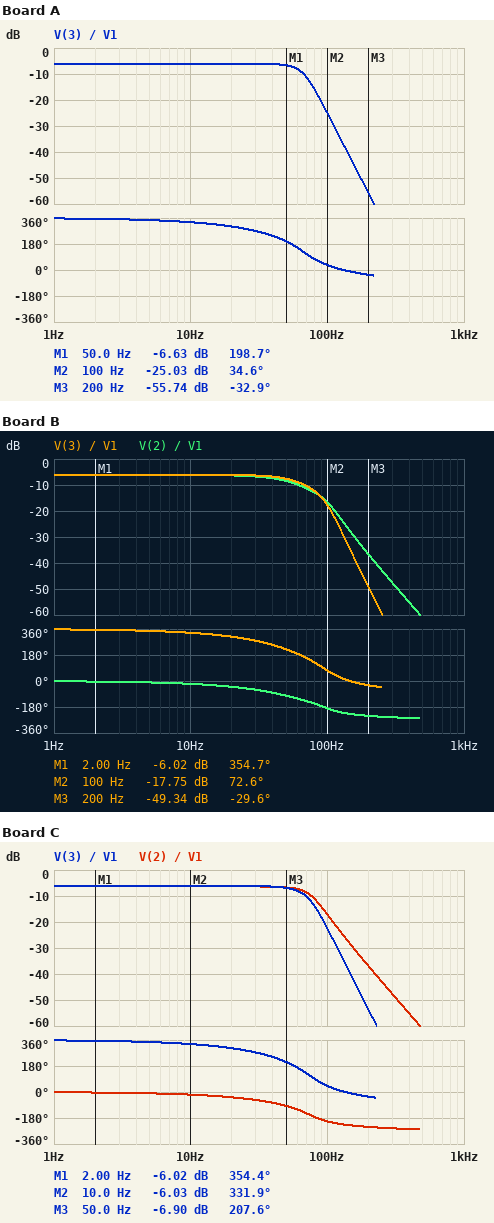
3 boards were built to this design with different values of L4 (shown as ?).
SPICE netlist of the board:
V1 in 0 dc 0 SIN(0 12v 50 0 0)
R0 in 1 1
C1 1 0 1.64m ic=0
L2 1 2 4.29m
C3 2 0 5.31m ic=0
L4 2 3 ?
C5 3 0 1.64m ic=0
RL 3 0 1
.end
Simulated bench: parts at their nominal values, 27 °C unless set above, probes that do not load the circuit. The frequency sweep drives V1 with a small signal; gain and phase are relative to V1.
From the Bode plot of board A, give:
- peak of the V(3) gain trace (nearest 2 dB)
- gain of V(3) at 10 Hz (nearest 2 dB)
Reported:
-6 dB
-6 dB
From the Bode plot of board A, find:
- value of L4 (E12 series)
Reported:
3.3 mH
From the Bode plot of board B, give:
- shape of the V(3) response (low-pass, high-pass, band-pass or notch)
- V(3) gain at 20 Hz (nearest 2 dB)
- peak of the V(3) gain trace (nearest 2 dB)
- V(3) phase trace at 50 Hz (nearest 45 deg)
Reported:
low-pass
-6 dB
-6 dB
225 deg
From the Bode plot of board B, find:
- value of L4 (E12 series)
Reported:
1.8 mH
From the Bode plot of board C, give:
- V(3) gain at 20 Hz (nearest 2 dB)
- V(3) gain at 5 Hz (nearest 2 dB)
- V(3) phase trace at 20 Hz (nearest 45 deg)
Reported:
-6 dB
-6 dB
315 deg
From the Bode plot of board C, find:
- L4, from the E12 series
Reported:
2.7 mH
